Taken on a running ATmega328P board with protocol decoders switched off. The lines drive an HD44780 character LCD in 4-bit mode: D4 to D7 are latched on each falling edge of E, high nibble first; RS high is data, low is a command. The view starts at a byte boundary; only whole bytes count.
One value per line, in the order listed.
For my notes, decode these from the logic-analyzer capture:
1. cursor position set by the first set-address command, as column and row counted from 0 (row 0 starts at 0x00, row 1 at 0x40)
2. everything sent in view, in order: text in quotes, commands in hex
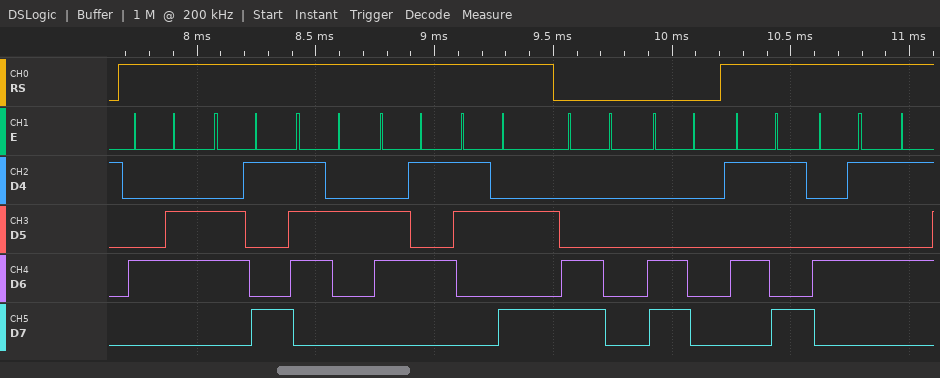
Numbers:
column 0, row 1
"Fire:" 0xC0 0xC0 "YE"
